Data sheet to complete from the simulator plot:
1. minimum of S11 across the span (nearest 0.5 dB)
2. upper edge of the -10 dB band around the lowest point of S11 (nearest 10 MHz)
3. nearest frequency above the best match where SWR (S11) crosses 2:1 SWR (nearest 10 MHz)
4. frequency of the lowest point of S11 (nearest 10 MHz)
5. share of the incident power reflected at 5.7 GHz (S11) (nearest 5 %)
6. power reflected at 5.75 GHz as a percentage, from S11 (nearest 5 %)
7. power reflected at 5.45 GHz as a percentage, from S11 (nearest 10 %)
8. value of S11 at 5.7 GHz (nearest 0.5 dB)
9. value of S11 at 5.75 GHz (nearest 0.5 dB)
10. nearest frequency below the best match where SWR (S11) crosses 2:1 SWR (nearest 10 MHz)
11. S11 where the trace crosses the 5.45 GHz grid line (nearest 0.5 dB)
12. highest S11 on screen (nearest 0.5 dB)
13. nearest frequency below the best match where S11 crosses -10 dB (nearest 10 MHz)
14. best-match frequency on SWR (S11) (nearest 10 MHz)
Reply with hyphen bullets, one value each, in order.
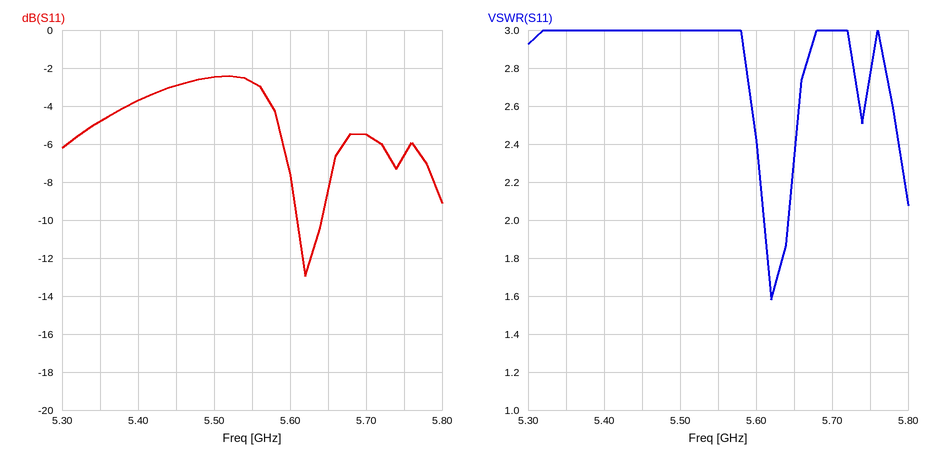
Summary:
- -13.0 dB
- 5.64 GHz
- 5.64 GHz
- 5.62 GHz
- 30 %
- 20 %
- 50 %
- -5.5 dB
- -6.5 dB
- 5.61 GHz
- -3.0 dB
- -2.5 dB
- 5.61 GHz
- 5.62 GHz
